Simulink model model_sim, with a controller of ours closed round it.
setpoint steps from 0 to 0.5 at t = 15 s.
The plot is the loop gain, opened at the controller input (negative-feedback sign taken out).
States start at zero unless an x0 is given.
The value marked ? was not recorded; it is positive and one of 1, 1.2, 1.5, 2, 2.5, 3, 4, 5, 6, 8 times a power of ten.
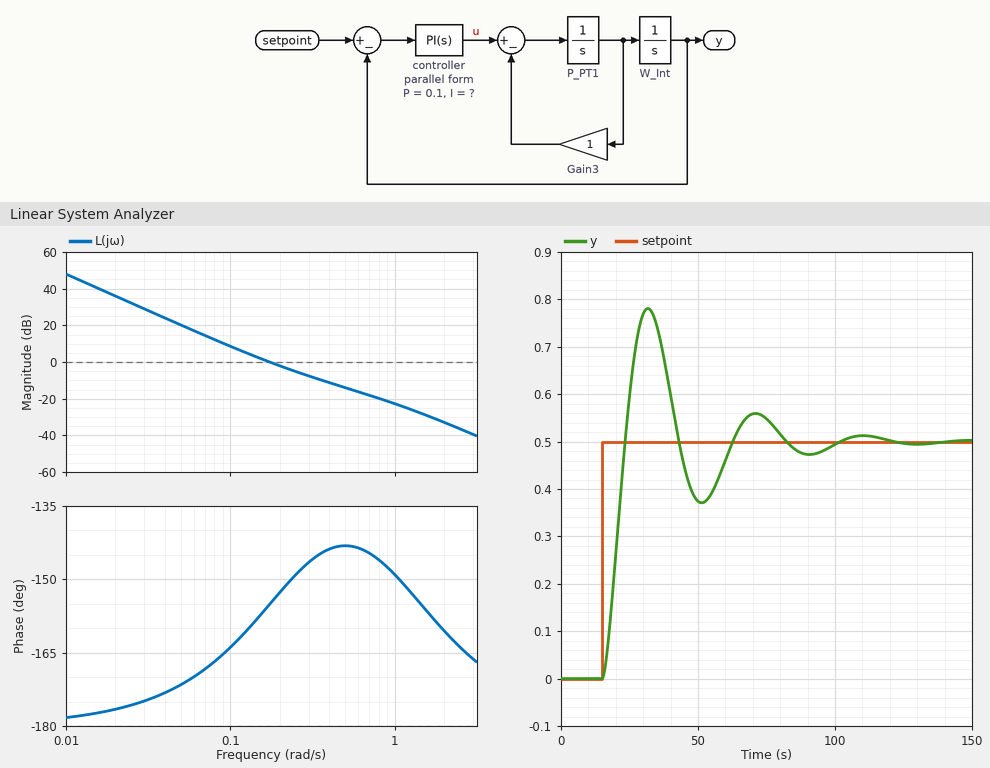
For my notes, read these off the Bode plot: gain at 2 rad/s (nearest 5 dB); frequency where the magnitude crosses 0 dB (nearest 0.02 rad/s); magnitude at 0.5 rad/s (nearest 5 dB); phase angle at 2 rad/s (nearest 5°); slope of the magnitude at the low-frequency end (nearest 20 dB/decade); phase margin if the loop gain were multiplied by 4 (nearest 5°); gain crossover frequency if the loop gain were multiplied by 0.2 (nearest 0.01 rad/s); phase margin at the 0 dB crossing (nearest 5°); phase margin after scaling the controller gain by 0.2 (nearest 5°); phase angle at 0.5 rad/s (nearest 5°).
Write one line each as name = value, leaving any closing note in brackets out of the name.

gain at 2 rad/s = -35 dB
frequency where the magnitude crosses 0 dB = 0.18 rad/s
magnitude at 0.5 rad/s = -15 dB
phase angle at 2 rad/s = -160°
slope of the magnitude at the low-frequency end = -40 dB/decade
phase margin if the loop gain were multiplied by 4 = 35°
gain crossover frequency if the loop gain were multiplied by 0.2 = 0.07 rad/s
phase margin at the 0 dB crossing = 25°
phase margin after scaling the controller gain by 0.2 = 10°
phase angle at 0.5 rad/s = -145°
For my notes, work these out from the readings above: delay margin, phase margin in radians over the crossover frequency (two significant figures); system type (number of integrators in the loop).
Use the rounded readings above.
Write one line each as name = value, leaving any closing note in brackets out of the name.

delay margin, phase margin in radians over the crossover frequency = 2.4 s
system type = 2
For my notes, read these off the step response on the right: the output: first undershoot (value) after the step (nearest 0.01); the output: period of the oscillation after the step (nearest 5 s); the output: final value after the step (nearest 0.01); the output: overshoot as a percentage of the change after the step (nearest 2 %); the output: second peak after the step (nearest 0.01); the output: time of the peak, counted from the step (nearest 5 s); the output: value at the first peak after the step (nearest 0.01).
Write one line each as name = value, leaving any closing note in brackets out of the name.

the output: first undershoot (value) after the step = 0.37
the output: period of the oscillation after the step = 40 s
the output: final value after the step = 0.50
the output: overshoot as a percentage of the change after the step = 56 %
the output: second peak after the step = 0.56
the output: time of the peak, counted from the step = 15 s
the output: value at the first peak after the step = 0.78
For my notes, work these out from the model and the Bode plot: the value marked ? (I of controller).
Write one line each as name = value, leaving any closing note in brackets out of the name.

the value marked ? = 0.025
